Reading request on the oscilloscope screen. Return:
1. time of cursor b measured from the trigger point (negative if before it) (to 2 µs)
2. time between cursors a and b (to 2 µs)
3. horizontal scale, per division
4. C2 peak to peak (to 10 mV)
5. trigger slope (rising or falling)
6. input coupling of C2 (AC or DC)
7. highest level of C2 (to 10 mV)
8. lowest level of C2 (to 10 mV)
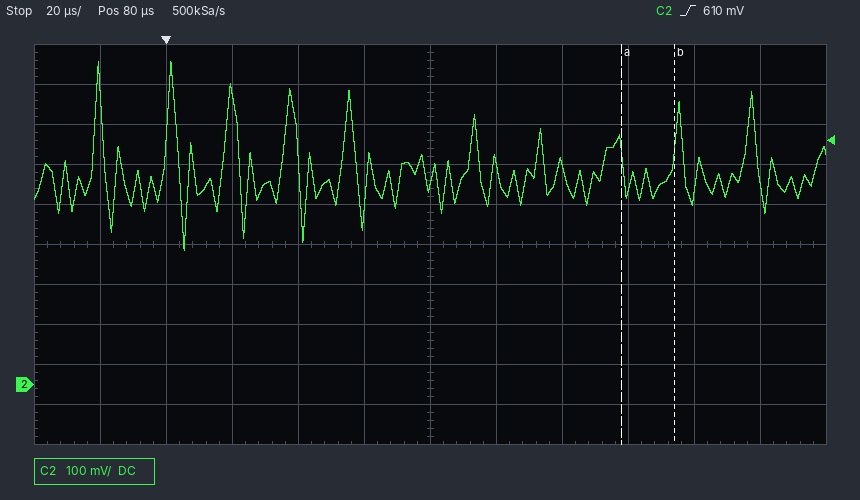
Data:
+154 µs
16 µs
20 µs
470 mV
rising
DC
810 mV
340 mV
